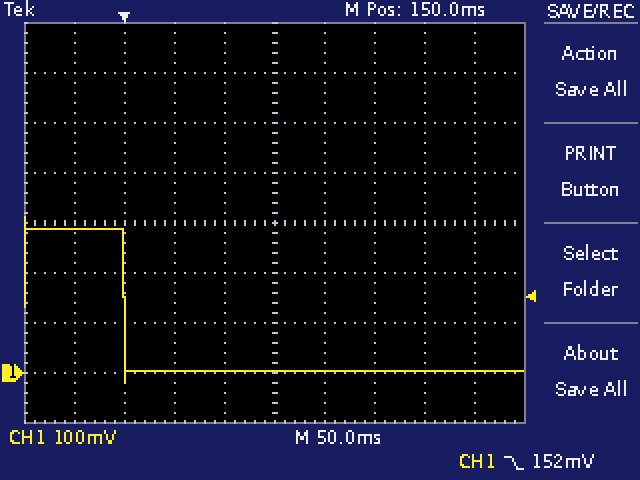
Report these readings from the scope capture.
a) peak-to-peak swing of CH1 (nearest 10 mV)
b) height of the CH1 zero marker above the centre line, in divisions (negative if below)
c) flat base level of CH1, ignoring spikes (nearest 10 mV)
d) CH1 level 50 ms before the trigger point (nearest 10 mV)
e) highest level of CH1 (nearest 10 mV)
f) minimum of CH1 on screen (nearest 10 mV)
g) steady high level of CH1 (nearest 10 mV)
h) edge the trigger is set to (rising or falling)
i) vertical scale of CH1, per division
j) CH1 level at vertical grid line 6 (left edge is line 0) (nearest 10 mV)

330 mV
-3.0 div
0 mV
290 mV
310 mV
-20 mV
290 mV
falling
100 mV
0 mV
